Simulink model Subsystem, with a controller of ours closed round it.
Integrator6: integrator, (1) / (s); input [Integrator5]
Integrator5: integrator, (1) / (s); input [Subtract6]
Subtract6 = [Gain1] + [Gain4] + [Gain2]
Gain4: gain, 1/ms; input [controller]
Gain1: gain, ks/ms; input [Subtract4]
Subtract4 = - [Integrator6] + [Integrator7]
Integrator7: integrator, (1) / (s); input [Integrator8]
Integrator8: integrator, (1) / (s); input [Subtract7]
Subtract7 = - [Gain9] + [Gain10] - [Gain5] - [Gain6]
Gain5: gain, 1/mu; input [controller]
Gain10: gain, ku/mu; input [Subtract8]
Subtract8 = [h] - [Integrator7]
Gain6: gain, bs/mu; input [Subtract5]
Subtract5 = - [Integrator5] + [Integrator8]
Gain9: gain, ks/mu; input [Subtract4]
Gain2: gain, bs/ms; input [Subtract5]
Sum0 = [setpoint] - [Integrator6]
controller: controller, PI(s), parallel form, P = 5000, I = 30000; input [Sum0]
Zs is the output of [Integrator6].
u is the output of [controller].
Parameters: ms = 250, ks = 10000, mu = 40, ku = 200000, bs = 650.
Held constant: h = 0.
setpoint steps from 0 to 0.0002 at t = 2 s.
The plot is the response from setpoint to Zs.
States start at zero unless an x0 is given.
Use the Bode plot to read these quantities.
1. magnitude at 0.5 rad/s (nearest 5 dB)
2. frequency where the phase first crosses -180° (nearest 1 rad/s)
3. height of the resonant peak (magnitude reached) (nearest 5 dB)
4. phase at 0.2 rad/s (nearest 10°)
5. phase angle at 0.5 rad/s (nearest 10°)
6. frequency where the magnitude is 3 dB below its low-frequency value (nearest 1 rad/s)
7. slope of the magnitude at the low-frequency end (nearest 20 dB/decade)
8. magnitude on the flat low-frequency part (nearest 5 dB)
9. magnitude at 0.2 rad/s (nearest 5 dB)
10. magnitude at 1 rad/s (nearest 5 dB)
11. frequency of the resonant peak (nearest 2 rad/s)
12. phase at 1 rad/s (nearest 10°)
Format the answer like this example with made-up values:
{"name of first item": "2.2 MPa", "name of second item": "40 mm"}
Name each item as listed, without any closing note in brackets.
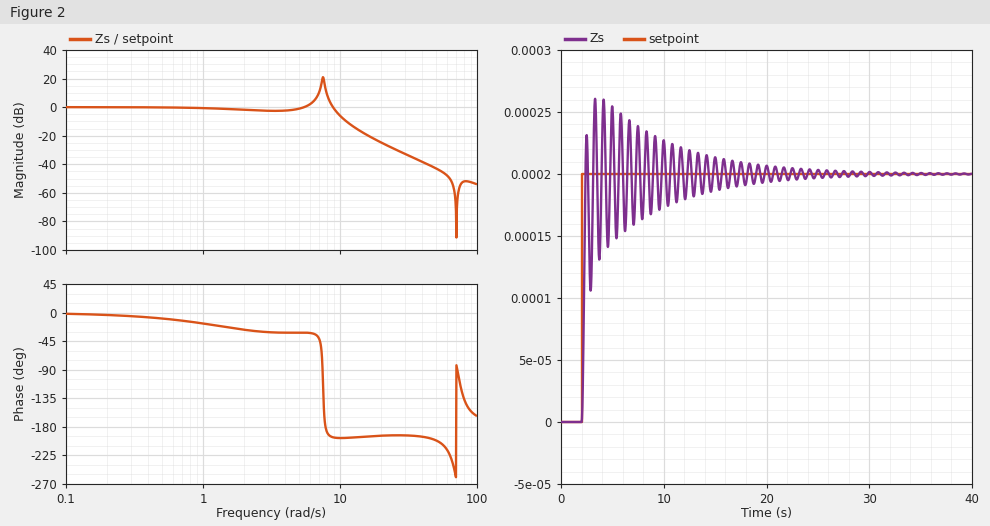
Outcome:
{"magnitude at 0.5 rad/s": "0 dB", "frequency where the phase first crosses -180°": "8 rad/s", "height of the resonant peak (magnitude reached)": "20 dB", "phase at 0.2 rad/s": "0°", "phase angle at 0.5 rad/s": "-10°", "frequency where the magnitude is 3 dB below its low-frequency value": "9 rad/s", "slope of the magnitude at the low-frequency end": "0 dB/decade", "magnitude on the flat low-frequency part": "0 dB", "magnitude at 0.2 rad/s": "0 dB", "magnitude at 1 rad/s": "0 dB", "frequency of the resonant peak": "8 rad/s", "phase at 1 rad/s": "-20°"}
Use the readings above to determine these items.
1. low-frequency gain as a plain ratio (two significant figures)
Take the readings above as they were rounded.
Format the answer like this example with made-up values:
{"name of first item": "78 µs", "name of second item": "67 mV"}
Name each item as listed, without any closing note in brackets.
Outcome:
{"low-frequency gain as a plain ratio": "1.0"}
